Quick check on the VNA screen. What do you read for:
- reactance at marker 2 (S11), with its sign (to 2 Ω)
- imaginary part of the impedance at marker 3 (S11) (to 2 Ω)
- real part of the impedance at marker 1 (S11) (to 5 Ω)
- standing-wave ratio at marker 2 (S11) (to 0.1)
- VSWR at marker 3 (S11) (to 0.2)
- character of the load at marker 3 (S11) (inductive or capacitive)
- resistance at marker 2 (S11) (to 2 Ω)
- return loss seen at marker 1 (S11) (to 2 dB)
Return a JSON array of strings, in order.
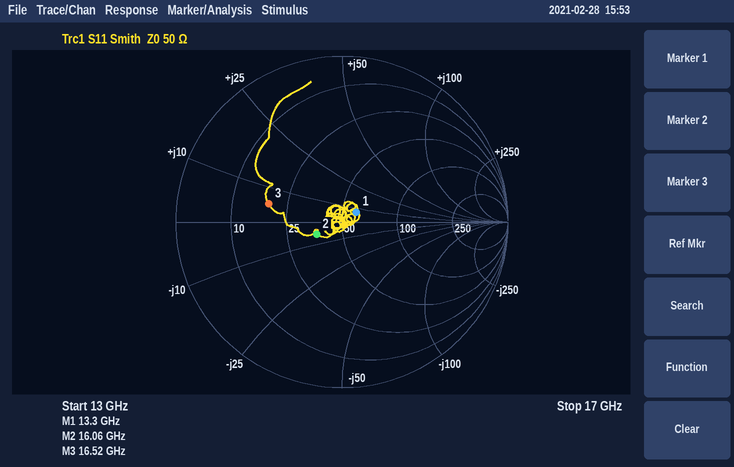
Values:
["-6 Ω", "+6 Ω", "60 Ω", "1.4", "2.6", "inductive", "36 Ω", "20 dB"]
